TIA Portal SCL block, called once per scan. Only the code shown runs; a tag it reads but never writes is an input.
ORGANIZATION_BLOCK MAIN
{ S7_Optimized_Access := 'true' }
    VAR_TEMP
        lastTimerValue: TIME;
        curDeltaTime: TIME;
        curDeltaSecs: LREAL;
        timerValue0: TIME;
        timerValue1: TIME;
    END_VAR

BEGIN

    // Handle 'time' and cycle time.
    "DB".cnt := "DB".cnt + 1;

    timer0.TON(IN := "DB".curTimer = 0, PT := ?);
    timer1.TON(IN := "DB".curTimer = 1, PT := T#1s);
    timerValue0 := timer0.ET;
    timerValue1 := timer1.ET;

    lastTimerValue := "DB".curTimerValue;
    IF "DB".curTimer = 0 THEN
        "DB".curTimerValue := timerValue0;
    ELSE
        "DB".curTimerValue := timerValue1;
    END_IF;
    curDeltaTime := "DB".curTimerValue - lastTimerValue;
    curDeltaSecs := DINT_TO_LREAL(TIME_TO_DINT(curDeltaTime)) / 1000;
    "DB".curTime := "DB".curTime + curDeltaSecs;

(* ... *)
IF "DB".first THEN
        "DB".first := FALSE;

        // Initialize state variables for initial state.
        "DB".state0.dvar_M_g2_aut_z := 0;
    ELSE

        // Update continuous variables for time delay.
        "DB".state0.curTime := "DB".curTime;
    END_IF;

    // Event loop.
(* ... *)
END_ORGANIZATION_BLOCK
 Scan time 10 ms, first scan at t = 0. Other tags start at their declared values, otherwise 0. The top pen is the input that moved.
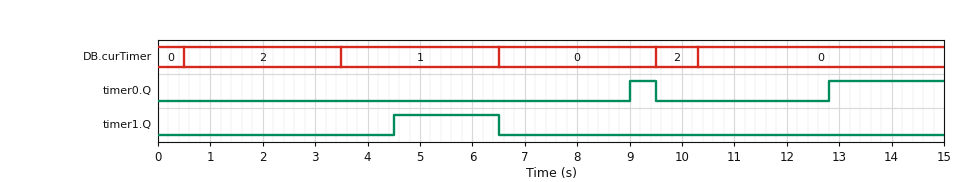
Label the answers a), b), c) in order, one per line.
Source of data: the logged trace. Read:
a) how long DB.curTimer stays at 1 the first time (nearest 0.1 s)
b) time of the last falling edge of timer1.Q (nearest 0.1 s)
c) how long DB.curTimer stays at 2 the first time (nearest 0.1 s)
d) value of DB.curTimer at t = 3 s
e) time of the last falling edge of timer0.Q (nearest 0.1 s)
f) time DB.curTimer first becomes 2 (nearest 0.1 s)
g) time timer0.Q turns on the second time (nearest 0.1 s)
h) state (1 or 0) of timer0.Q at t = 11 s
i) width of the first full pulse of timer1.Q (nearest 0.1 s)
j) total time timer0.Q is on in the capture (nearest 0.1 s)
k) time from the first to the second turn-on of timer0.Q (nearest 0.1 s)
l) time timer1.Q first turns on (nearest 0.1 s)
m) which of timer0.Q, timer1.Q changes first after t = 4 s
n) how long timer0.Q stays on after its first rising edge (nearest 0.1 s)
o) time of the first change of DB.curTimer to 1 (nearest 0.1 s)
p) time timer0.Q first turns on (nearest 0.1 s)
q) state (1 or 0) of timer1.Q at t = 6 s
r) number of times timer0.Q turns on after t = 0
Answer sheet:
a) 3.0 s
b) 6.5 s
c) 3.0 s
d) 2
e) 9.5 s
f) 0.5 s
g) 12.8 s
h) 0
i) 2.0 s
j) 2.7 s
k) 3.8 s
l) 4.5 s
m) timer1.Q
n) 0.5 s
o) 3.5 s
p) 9.0 s
q) 1
r) 2
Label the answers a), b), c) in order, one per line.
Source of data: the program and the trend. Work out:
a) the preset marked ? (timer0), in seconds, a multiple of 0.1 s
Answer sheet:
a) 2.5 s
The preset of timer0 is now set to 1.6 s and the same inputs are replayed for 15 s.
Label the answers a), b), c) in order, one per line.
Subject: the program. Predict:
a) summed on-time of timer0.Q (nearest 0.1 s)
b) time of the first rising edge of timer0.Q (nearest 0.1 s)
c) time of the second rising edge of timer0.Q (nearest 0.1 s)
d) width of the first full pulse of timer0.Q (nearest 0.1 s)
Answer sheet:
a) 4.5 s
b) 8.1 s
c) 11.9 s
d) 1.4 s
